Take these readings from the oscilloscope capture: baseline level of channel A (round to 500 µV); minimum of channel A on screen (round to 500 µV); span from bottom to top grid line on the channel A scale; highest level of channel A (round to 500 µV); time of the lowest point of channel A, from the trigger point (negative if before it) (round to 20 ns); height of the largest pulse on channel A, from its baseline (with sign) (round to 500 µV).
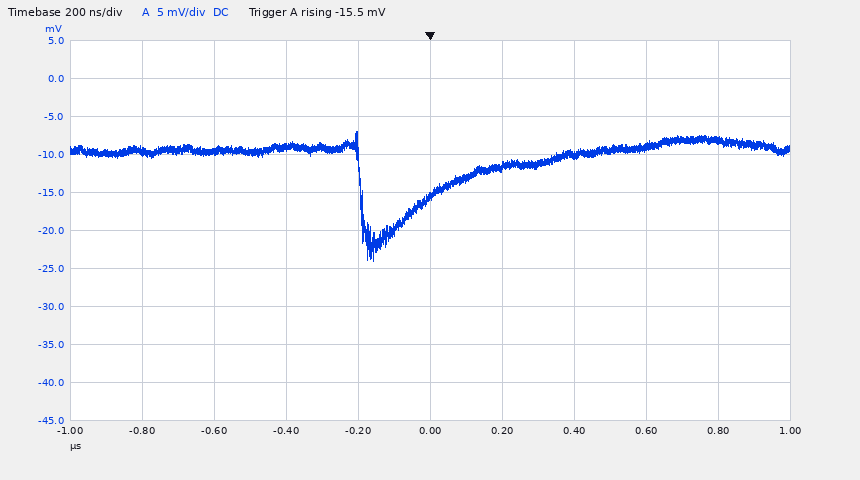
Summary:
-9.5 mV
-24.0 mV
50 mV
-7.0 mV
-160 ns
-14.5 mV
